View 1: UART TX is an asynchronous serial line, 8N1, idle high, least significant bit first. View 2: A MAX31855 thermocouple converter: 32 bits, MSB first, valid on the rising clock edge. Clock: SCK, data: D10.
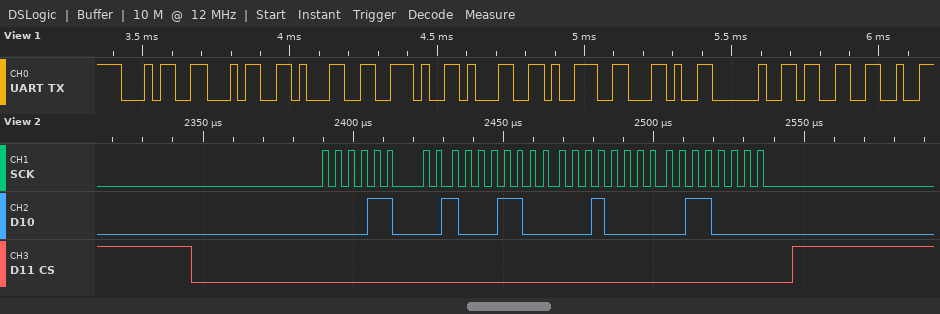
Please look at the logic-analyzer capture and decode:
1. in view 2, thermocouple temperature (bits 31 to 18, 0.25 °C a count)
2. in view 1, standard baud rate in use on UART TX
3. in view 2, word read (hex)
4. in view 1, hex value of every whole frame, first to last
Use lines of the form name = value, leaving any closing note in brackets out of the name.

in view 2, thermocouple temperature = 200.75 °C
in view 1, standard baud rate in use on UART TX = 38400 baud
in view 2, word read = 0x0C8C1030
in view 1, hex value of every whole frame, first to last = 34 34 31 2E 31 39 2C 20 33
